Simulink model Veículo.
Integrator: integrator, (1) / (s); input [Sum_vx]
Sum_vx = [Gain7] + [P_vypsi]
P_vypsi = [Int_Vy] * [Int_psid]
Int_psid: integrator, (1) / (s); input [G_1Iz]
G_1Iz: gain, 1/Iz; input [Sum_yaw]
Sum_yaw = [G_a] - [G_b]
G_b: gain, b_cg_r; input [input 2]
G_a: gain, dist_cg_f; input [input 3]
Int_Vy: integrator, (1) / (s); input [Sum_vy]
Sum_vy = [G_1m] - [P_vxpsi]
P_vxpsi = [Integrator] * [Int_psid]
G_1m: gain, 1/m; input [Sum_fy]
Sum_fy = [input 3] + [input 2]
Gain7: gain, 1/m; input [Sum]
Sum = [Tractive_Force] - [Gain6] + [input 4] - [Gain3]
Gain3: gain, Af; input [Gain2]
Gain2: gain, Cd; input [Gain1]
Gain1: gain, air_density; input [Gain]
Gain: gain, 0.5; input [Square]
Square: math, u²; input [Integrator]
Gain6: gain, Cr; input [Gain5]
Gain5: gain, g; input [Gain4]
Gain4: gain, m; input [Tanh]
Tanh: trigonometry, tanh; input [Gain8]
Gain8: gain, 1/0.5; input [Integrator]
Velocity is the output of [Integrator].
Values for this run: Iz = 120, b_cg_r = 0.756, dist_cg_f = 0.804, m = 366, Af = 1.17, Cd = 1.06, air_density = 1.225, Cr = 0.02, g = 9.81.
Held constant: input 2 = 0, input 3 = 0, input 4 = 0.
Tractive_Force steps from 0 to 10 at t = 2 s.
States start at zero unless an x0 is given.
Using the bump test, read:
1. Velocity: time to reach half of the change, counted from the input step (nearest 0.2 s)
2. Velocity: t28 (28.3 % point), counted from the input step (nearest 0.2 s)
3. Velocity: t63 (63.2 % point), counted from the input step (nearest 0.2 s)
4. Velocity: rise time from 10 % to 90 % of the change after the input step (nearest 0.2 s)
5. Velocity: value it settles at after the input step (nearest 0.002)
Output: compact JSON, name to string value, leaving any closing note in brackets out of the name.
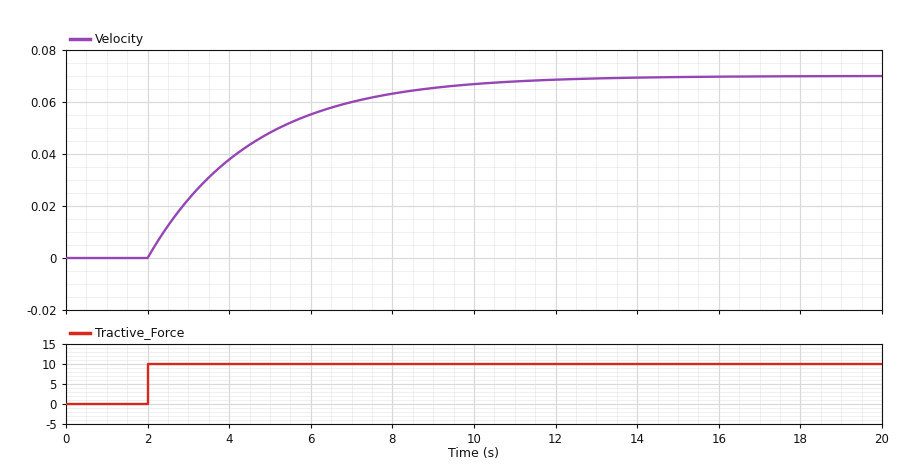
{"Velocity: time to reach half of the change, counted from the input step": "1.8 s", "Velocity: t28 (28.3 % point), counted from the input step": "0.8 s", "Velocity: t63 (63.2 % point), counted from the input step": "2.6 s", "Velocity: rise time from 10 % to 90 % of the change after the input step": "5.6 s", "Velocity: value it settles at after the input step": "0.070"}
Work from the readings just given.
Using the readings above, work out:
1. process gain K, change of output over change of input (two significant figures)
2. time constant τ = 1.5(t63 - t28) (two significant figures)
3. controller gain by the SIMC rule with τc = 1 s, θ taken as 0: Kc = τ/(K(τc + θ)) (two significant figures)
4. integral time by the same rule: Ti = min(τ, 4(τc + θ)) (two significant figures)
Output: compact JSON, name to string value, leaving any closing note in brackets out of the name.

{"process gain K, change of output over change of input": "0.0070", "time constant τ = 1.5(t63 - t28)": "2.7 s", "controller gain by the SIMC rule with τc = 1 s, θ taken as 0: Kc = τ/(K(τc + θ))": "390", "integral time by the same rule: Ti = min(τ, 4(τc + θ))": "2.7 s"}
